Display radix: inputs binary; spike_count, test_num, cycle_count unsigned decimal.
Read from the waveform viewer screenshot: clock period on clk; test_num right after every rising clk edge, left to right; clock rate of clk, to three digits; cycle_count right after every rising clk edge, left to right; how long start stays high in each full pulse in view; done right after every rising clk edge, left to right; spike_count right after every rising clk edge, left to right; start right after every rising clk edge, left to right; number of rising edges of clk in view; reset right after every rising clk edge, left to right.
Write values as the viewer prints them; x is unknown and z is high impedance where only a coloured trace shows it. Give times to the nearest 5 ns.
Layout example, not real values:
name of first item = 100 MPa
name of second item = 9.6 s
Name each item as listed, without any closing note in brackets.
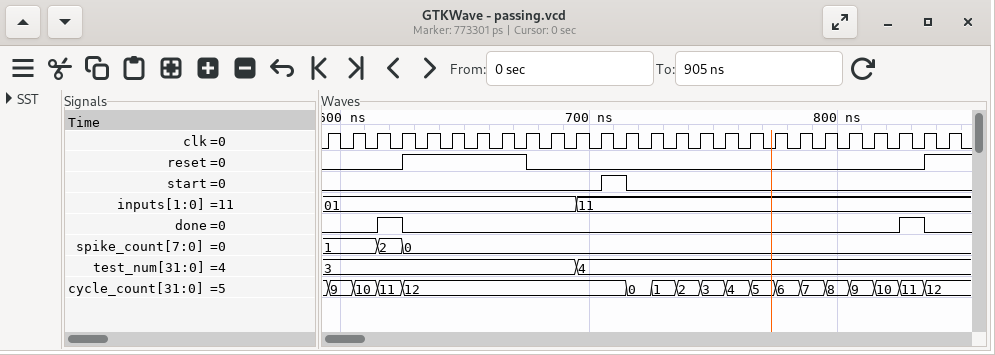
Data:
clock period on clk = 10 ns
test_num right after every rising clk edge, left to right = 3, 3, 3, 3, 3, 3, 3, 3, 3, 3, 4, 4, 4, 4, 4, 4, 4, 4, 4, 4, 4, 4, 4, 4, 4, 4
clock rate of clk, to three digits = 100 MHz
cycle_count right after every rising clk edge, left to right = 9, 10, 11, 12, 12, 12, 12, 12, 12, 12, 12, 12, 0, 1, 2, 3, 4, 5, 6, 7, 8, 9, 10, 11, 12, 12
how long start stays high in each full pulse in view = 10 ns
done right after every rising clk edge, left to right = 0 0 1 0 0 0 0 0 0 0 0 0 0 0 0 0 0 0 0 0 0 0 0 1 0 0
spike_count right after every rising clk edge, left to right = 1, 1, 2, 0, 0, 0, 0, 0, 0, 0, 0, 0, 0, 0, 0, 0, 0, 0, 0, 0, 0, 0, 0, 0, 0, 0
start right after every rising clk edge, left to right = 0 0 0 0 0 0 0 0 0 0 0 1 0 0 0 0 0 0 0 0 0 0 0 0 0 0
number of rising edges of clk in view = 26
reset right after every rising clk edge, left to right = 0 0 0 1 1 1 1 1 0 0 0 0 0 0 0 0 0 0 0 0 0 0 0 0 1 1
